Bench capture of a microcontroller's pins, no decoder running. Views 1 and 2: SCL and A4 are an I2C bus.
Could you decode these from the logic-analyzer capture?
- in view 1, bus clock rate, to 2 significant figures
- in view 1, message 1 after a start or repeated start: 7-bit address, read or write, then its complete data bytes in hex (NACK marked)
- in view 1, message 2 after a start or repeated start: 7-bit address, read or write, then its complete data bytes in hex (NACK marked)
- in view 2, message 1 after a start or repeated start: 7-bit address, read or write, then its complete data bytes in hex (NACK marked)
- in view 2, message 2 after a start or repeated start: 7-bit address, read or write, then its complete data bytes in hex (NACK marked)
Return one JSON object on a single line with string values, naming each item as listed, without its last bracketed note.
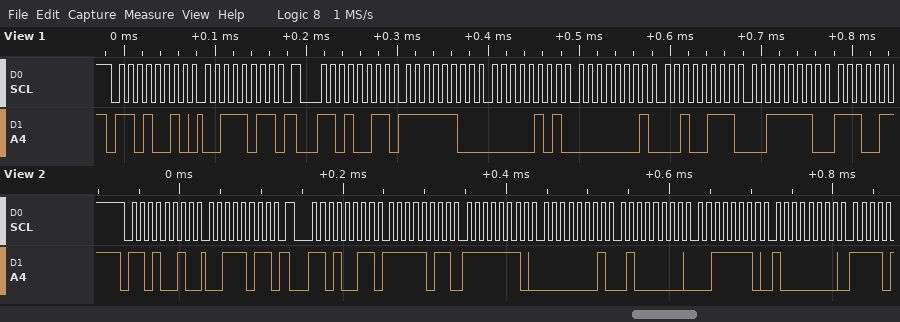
{"in view 1, bus clock rate, to 2 significant figures": "100 kHz", "in view 1, message 1 after a start or repeated start: 7-bit address, read or write, then its complete data bytes in hex": "0x69 write: 3B", "in view 1, message 2 after a start or repeated start: 7-bit address, read or write, then its complete data bytes in hex": "0x69 read: FC 05 01 27 3E", "in view 2, message 1 after a start or repeated start: 7-bit address, read or write, then its complete data bytes in hex": "0x69 write: 3B", "in view 2, message 2 after a start or repeated start: 7-bit address, read or write, then its complete data bytes in hex": "0x69 read: FB FE 01 40 3E 80"}
